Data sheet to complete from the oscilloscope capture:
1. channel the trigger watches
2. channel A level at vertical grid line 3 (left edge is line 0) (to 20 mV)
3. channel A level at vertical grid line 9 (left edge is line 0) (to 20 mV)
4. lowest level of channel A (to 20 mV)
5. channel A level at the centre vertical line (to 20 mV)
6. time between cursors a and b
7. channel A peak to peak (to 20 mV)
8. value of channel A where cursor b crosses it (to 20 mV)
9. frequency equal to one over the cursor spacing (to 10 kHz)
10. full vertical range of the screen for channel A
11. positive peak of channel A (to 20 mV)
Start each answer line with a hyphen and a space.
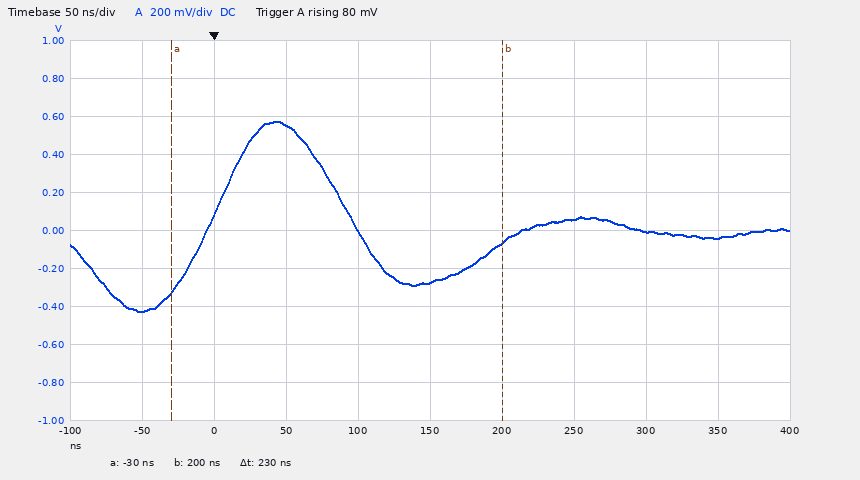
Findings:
- channel A
- 560 mV
- -40 mV
- -420 mV
- -280 mV
- 230 ns
- 1.00 V
- -60 mV
- 4.35 MHz
- 2 V
- 580 mV
